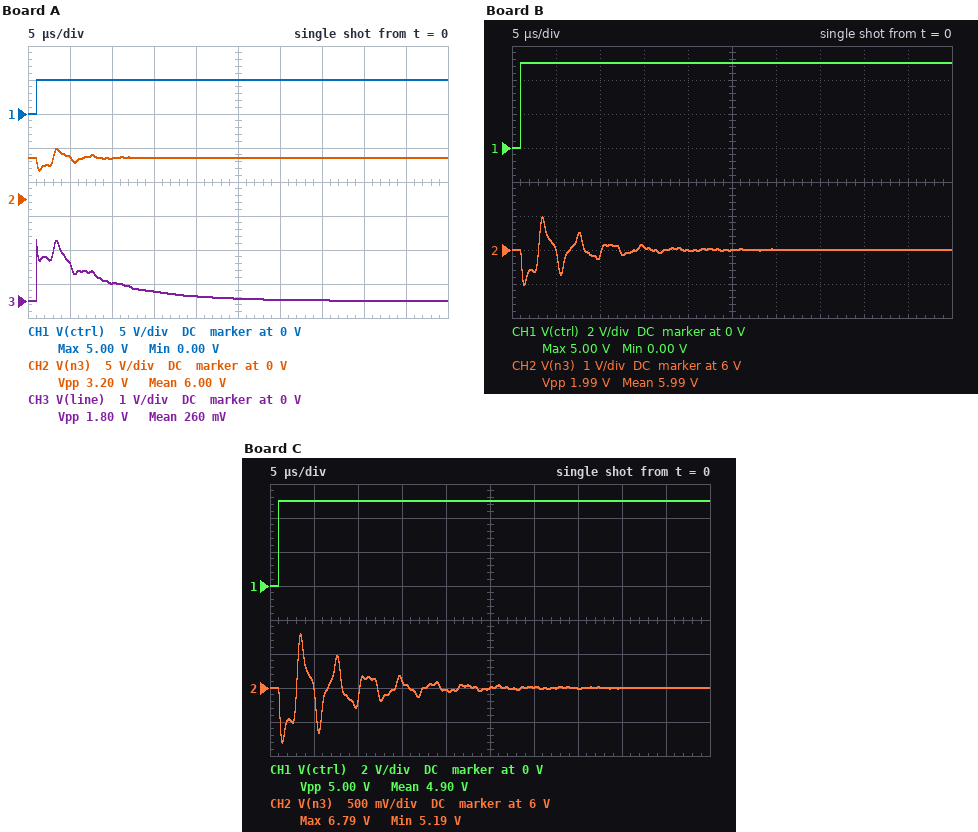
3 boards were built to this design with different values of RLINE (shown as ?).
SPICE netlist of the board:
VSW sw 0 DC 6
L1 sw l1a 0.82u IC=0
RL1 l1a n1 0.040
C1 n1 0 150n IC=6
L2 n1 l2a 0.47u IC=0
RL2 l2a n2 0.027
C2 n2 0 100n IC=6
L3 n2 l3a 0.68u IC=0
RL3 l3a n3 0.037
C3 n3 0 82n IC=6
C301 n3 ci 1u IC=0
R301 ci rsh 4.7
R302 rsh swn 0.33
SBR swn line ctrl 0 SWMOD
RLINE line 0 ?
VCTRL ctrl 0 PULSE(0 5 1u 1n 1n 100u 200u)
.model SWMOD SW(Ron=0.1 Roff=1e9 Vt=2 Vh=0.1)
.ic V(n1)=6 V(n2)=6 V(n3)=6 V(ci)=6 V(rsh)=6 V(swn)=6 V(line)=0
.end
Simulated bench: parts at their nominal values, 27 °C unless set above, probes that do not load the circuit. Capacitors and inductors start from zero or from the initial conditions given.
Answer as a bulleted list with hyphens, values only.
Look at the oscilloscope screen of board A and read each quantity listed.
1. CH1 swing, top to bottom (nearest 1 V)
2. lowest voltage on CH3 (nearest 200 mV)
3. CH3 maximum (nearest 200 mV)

- 5 V
- 0 V
- 1.8 V
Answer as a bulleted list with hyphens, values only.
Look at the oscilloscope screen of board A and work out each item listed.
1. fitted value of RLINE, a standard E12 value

- 2.2 Ω
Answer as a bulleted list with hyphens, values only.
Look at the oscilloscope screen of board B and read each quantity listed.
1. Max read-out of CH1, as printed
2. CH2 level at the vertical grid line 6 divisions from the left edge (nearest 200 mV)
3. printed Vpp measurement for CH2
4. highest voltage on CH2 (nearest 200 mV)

- 5.00 V
- 6.0 V
- 1.99 V
- 7.0 V
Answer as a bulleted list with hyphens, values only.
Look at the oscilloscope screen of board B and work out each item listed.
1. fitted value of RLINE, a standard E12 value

- 10 Ω
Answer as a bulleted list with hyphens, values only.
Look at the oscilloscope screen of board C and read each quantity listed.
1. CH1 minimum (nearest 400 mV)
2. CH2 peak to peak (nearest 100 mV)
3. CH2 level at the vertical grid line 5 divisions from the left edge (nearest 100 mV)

- 0 V
- 1.6 V
- 6.0 V
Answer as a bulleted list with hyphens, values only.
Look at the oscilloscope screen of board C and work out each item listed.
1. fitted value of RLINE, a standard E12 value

- 15 Ω
